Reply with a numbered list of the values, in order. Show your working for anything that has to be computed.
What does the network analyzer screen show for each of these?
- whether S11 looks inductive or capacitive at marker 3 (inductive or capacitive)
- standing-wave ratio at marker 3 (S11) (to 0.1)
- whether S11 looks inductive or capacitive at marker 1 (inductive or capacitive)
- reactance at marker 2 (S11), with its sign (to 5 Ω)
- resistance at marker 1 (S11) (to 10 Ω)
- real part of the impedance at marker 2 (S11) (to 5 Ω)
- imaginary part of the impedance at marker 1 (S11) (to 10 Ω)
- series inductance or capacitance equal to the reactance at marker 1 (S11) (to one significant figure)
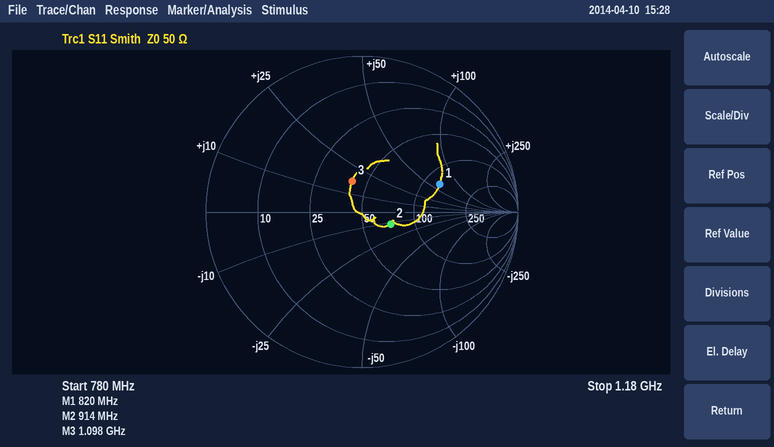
1. inductive
2. 1.5
3. inductive
4. -10 Ω
5. 130 Ω
6. 70 Ω
7. +60 Ω
8. L = 60 Ω/(2π × 820 MHz) ≈ 11.6 nH, so 10 nH to one significant figure
